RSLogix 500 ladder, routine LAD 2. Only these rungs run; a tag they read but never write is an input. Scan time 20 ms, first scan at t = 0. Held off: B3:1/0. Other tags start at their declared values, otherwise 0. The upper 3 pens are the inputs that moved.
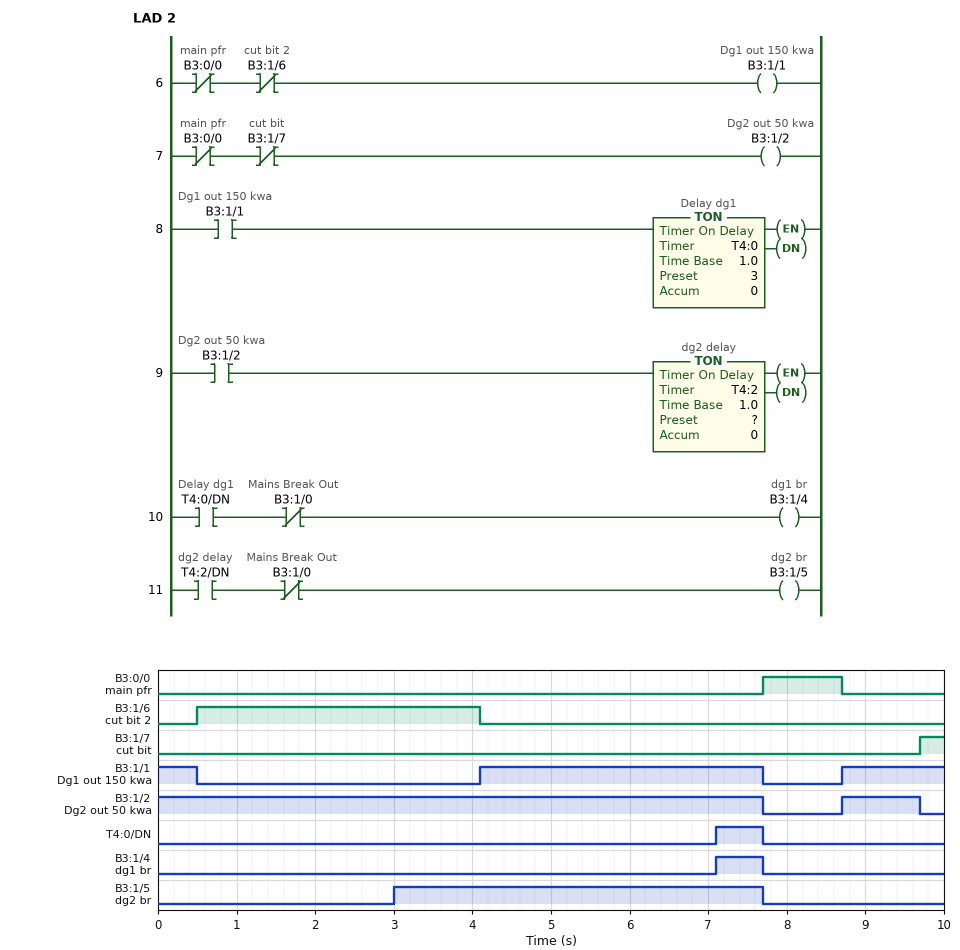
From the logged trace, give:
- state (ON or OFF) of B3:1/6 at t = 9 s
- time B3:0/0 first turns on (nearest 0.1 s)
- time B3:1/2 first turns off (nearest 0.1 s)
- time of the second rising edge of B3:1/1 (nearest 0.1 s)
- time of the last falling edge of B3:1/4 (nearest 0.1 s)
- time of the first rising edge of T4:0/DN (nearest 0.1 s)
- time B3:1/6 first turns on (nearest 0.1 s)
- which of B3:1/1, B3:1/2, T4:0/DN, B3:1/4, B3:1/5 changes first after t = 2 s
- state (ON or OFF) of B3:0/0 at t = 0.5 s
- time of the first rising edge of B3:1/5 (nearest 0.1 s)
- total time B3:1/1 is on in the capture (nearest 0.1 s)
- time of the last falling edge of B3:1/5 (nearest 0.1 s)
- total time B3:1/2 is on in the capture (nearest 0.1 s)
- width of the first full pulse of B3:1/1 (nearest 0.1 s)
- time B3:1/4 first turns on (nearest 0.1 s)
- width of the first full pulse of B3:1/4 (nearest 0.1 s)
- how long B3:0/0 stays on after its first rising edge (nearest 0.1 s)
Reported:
OFF
7.7 s
7.7 s
8.7 s
7.7 s
7.1 s
0.5 s
B3:1/5
OFF
3.0 s
5.4 s
7.7 s
8.7 s
3.6 s
7.1 s
0.6 s
1.0 s
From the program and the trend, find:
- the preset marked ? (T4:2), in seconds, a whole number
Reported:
3 s
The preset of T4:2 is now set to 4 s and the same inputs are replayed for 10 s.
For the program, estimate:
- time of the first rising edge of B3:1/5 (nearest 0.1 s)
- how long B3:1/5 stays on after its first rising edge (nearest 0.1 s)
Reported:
4.0 s
3.7 s
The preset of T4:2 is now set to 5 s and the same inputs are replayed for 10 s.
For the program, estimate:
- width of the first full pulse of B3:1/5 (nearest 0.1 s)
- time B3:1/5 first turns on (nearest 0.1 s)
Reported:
2.7 s
5.0 s
